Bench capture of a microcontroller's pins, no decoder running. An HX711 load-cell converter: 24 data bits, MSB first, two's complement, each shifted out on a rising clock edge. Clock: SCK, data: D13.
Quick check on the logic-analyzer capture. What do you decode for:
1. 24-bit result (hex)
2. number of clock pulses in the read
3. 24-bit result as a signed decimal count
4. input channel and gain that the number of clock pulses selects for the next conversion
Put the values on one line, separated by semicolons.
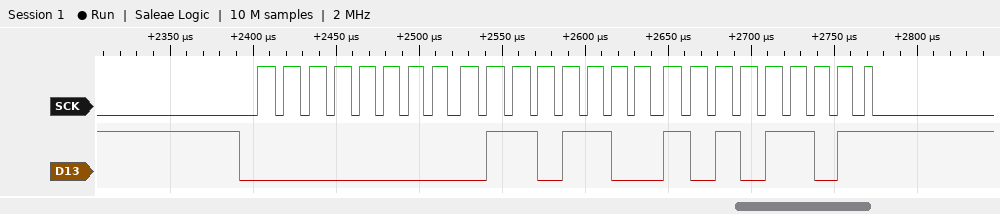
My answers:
0x006CAD; 25; 27821; channel A, gain 128
